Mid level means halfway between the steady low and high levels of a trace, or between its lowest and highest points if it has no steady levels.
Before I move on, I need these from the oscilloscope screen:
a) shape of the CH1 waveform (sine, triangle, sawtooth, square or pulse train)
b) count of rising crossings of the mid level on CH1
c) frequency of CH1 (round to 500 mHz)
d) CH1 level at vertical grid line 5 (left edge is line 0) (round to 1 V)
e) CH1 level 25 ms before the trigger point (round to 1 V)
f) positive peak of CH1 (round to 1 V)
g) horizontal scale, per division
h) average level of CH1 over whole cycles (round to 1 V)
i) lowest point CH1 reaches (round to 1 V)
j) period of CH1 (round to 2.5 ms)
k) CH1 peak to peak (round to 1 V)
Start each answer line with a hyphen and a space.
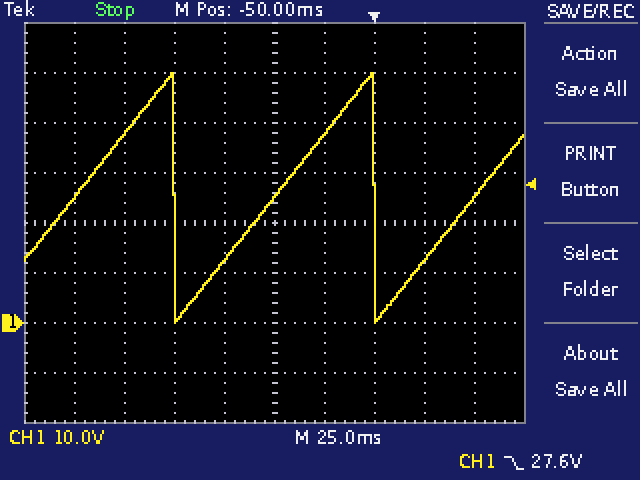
- sawtooth
- 3
- 10.0 Hz
- 25 V
- 38 V
- 50 V
- 25 ms
- 25 V
- 0 V
- 100.0 ms
- 50 V
